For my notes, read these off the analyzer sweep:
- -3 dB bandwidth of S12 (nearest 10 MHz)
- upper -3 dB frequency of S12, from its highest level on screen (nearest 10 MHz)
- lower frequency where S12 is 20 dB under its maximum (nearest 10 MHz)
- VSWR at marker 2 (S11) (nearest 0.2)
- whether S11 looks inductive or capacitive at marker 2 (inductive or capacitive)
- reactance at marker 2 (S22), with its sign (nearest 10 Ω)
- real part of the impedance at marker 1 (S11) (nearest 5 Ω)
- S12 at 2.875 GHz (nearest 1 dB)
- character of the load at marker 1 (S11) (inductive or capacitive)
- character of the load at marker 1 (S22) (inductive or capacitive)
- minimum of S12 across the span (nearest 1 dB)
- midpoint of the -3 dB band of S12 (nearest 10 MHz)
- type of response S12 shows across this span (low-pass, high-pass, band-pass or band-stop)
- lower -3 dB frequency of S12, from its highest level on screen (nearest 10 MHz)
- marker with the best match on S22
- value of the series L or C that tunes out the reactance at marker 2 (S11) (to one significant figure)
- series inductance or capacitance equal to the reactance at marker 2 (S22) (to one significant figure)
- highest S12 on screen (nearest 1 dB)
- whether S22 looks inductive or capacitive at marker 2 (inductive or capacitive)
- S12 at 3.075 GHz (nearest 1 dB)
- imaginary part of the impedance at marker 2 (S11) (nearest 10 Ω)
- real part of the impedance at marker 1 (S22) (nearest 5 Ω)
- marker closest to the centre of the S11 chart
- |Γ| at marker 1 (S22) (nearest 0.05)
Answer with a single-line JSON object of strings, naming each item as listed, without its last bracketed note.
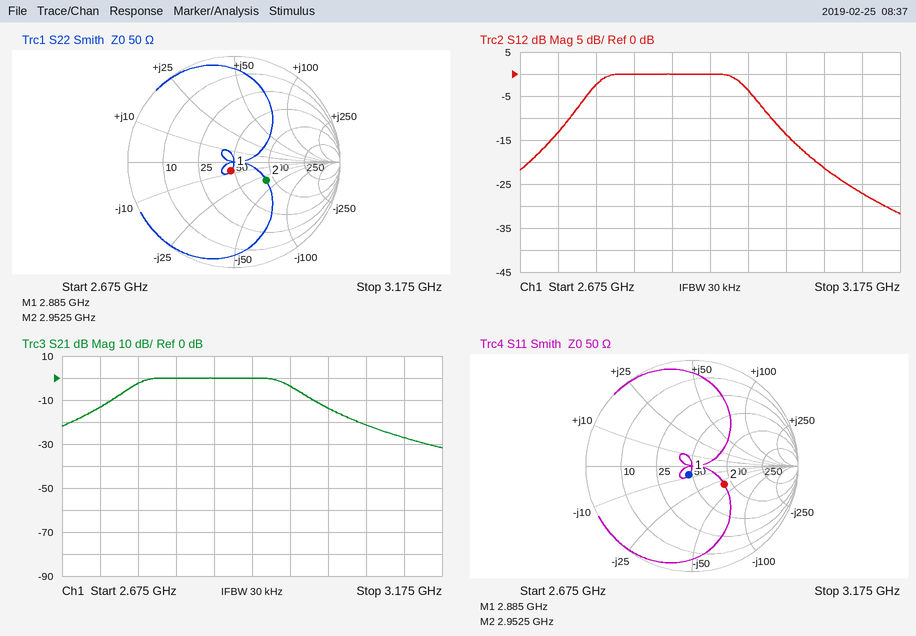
{"-3 dB bandwidth of S12": "200 MHz", "upper -3 dB frequency of S12, from its highest level on screen": "2.97 GHz", "lower frequency where S12 is 20 dB under its maximum": "2.69 GHz", "VSWR at marker 2 (S11)": "2.0", "whether S11 looks inductive or capacitive at marker 2": "capacitive", "reactance at marker 2 (S22), with its sign": "-30 Ω", "real part of the impedance at marker 1 (S11)": "45 Ω", "S12 at 2.875 GHz": "0 dB", "character of the load at marker 1 (S11)": "capacitive", "character of the load at marker 1 (S22)": "capacitive", "minimum of S12 across the span": "-32 dB", "midpoint of the -3 dB band of S12": "2.87 GHz", "type of response S12 shows across this span": "band-pass", "lower -3 dB frequency of S12, from its highest level on screen": "2.77 GHz", "marker with the best match on S22": "marker 1", "value of the series L or C that tunes out the reactance at marker 2 (S11)": "2 nH", "series inductance or capacitance equal to the reactance at marker 2 (S22)": "2 pF", "highest S12 on screen": "0 dB", "whether S22 looks inductive or capacitive at marker 2": "capacitive", "S12 at 3.075 GHz": "-21 dB", "imaginary part of the impedance at marker 2 (S11)": "-30 Ω", "real part of the impedance at marker 1 (S22)": "45 Ω", "marker closest to the centre of the S11 chart": "marker 1", "|Γ| at marker 1 (S22)": "0.10"}
